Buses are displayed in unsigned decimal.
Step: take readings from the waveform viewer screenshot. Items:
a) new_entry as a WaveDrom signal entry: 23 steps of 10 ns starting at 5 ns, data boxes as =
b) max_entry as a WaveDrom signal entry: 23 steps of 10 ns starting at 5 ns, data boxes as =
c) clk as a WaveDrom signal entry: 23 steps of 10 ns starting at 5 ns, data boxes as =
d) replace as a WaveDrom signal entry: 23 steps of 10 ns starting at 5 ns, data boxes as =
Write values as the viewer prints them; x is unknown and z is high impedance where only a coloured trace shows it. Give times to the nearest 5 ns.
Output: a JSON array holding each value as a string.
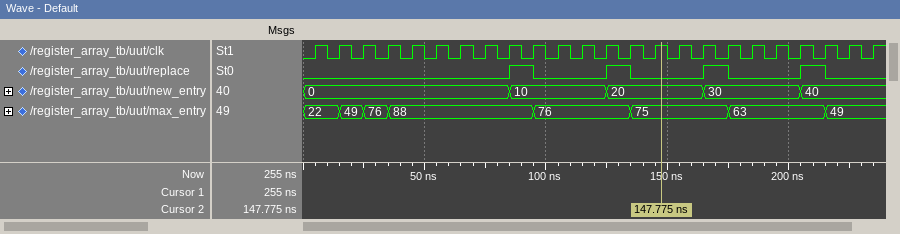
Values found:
["{name: 'new_entry', wave: '=.......=...=...=...=..', data: '0 10 20 30 40'}", "{name: 'max_entry', wave: '====.....=...=...=...=.', data: '22 49 76 88 76 75 63 49'}", "{name: 'clk', wave: 'p......................'}", "{name: 'replace', wave: '0.......10..10..10..10.'}"]
